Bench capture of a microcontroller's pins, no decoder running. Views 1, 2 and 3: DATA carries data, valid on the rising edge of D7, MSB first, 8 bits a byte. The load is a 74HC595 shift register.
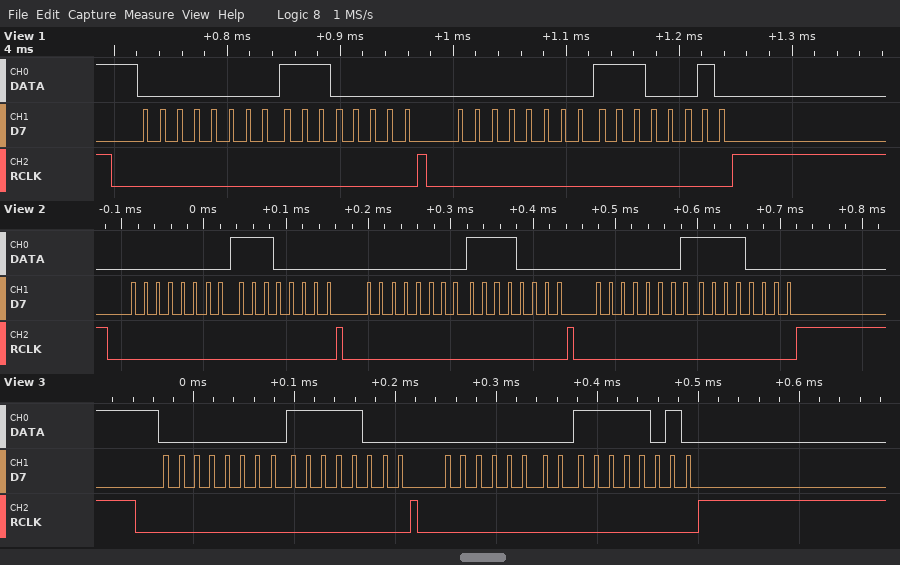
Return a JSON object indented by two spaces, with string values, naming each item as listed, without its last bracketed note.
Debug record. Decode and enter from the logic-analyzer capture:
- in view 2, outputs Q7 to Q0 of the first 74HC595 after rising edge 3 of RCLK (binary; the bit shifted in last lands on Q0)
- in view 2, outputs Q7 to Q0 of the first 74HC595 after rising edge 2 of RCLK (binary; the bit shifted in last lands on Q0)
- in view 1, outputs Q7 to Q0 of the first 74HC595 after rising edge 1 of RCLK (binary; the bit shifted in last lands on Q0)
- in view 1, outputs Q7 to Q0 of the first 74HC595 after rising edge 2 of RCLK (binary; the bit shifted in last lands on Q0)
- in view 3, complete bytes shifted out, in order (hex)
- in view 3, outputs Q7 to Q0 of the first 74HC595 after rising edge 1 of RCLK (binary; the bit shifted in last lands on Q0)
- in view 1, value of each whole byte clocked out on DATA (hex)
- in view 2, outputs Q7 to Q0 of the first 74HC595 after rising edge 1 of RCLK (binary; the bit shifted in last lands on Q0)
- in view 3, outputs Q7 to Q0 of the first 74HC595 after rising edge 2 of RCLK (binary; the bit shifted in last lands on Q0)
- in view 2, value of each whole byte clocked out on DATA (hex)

{
  "in view 2, outputs Q7 to Q0 of the first 74HC595 after rising edge 3 of RCLK": "11110000",
  "in view 2, outputs Q7 to Q0 of the first 74HC595 after rising edge 2 of RCLK": "11110000",
  "in view 1, outputs Q7 to Q0 of the first 74HC595 after rising edge 1 of RCLK": "11100000",
  "in view 1, outputs Q7 to Q0 of the first 74HC595 after rising edge 2 of RCLK": "11100010",
  "in view 3, complete bytes shifted out, in order": "00 F8 00 FA",
  "in view 3, outputs Q7 to Q0 of the first 74HC595 after rising edge 1 of RCLK": "11111000",
  "in view 1, value of each whole byte clocked out on DATA": "0x00 0xE0 0x00 0xE2",
  "in view 2, outputs Q7 to Q0 of the first 74HC595 after rising edge 1 of RCLK": "11100000",
  "in view 3, outputs Q7 to Q0 of the first 74HC595 after rising edge 2 of RCLK": "11111010",
  "in view 2, value of each whole byte clocked out on DATA": "00 E0 00 F0 01 F0"
}
